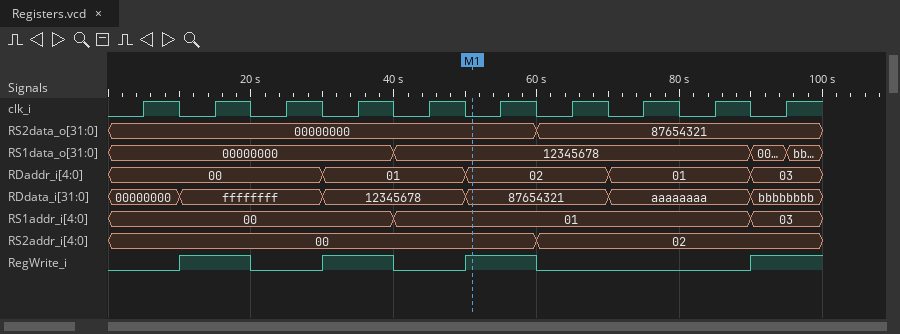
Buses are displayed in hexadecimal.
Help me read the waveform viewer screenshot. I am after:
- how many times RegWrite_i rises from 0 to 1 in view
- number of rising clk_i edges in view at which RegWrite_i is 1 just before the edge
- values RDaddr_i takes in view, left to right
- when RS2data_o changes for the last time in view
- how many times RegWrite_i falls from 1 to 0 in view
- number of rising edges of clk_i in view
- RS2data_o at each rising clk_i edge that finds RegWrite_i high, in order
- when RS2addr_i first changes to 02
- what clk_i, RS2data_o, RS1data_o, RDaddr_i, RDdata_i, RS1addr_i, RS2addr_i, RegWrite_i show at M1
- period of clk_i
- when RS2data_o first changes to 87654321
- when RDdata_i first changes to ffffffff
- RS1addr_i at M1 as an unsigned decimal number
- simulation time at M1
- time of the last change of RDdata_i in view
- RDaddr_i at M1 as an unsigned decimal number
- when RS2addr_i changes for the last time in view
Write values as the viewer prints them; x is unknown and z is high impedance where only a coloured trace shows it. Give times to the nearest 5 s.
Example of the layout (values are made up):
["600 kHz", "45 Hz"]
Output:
["4", "4", "00, 01, 02, 01, 03", "60 s", "3", "10", "00000000, 00000000, 00000000, 87654321", "60 s", "clk_i=0, RS2data_o=00000000, RS1data_o=12345678, RDaddr_i=02, RDdata_i=87654321, RS1addr_i=01, RS2addr_i=00, RegWrite_i=1", "10 s", "60 s", "10 s", "1", "50 s", "90 s", "2", "60 s"]
